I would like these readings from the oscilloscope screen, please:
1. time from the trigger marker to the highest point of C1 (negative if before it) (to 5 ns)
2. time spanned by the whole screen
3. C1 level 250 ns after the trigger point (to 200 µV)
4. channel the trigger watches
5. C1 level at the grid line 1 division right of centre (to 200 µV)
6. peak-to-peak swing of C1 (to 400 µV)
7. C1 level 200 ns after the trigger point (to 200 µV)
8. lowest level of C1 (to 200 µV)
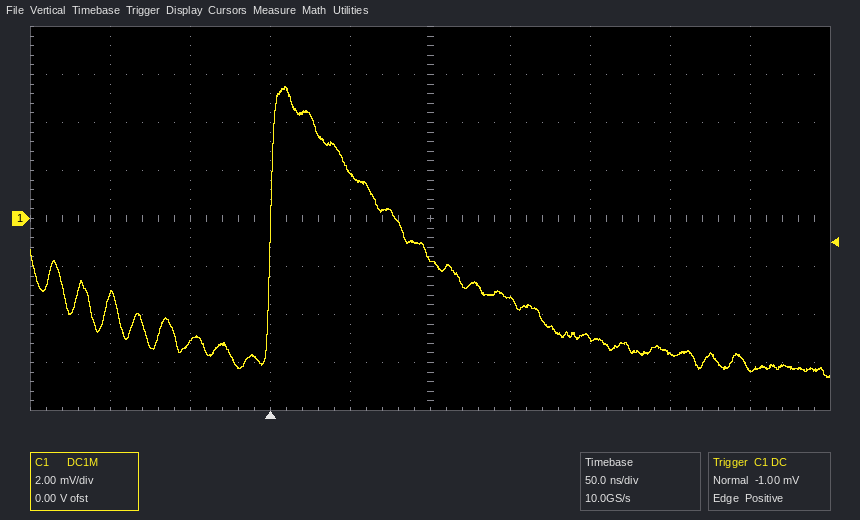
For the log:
+10 ns
500 ns
-5.6 mV
C1
-3.4 mV
12.0 mV
-5.0 mV
-6.6 mV
